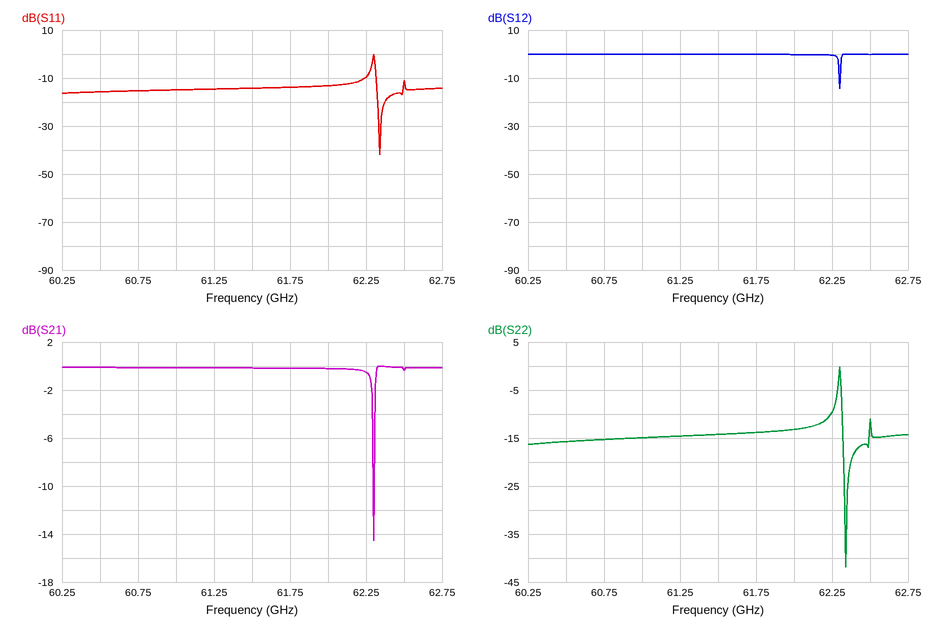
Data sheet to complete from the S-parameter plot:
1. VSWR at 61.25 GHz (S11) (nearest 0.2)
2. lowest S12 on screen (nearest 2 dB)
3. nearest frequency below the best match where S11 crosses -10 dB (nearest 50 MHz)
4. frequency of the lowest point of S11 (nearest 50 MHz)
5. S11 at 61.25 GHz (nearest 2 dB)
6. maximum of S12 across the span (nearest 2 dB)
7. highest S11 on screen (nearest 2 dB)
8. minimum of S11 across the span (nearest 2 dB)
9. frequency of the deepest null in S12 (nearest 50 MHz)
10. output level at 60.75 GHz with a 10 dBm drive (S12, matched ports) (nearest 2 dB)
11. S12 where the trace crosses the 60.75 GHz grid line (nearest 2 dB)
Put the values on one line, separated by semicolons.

1.4; -14 dB; 62.30 GHz; 62.35 GHz; -14 dB; 0 dB; 0 dB; -42 dB; 62.30 GHz; 10 dBm; 0 dB
